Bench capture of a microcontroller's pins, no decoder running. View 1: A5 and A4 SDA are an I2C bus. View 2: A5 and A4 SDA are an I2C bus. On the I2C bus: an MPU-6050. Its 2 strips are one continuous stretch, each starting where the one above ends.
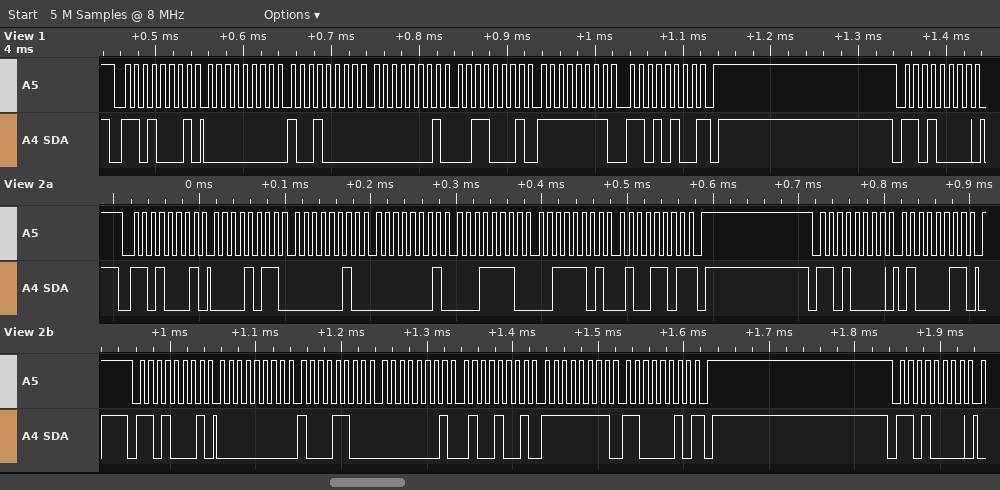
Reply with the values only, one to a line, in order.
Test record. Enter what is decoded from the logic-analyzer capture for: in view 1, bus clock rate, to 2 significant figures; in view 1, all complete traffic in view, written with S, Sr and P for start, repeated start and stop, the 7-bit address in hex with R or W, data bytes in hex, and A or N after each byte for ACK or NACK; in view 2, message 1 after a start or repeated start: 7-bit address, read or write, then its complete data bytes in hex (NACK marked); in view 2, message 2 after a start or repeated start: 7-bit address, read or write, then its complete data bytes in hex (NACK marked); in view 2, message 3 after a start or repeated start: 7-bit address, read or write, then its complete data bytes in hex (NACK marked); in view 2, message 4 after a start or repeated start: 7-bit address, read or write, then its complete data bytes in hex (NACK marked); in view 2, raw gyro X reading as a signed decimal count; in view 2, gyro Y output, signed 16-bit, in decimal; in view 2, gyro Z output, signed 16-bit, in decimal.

100 kHz
S 68R A 00 A 90 A 01 A 31 A FF A D4 N P S 68W A
0x68 read: 0B 02 01 1E 3D 4D NACK
0x68 write: 43
0x68 read: 00 8C 01 49 FF C2 NACK
0x68 write
140
329
-62
